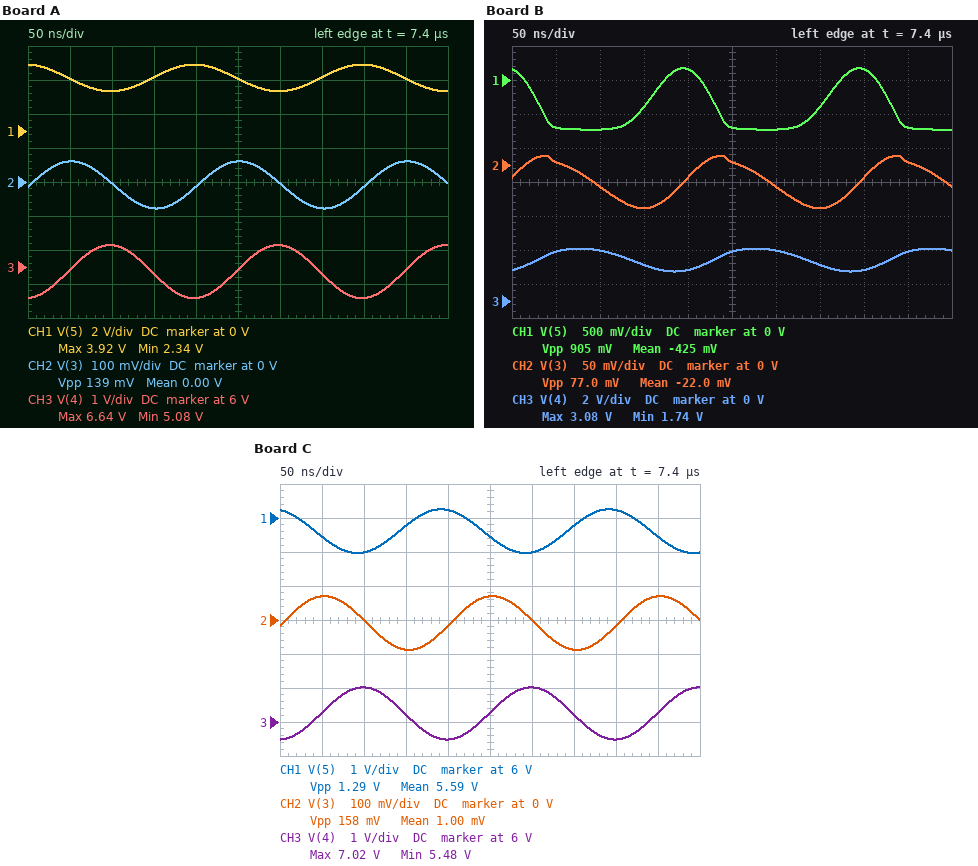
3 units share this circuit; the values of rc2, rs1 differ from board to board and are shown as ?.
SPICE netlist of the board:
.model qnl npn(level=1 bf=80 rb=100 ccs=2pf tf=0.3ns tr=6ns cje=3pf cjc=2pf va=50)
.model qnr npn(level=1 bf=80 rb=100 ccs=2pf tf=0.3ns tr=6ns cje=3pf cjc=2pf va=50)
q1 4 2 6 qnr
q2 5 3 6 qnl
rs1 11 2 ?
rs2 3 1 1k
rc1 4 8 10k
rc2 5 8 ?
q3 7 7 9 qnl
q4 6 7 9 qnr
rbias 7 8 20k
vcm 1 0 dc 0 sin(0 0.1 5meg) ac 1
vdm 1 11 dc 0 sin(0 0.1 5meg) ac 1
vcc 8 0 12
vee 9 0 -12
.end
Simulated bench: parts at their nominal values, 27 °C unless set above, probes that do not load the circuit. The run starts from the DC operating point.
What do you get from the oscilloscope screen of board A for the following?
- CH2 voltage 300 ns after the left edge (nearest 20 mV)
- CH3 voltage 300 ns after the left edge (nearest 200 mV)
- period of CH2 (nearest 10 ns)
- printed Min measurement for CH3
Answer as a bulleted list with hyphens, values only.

- 0 V
- 6.6 V
- 200 ns
- 5.08 V
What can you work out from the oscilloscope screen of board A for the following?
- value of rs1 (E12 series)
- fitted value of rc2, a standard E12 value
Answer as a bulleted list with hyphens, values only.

- 2.2 kΩ
- 12 kΩ
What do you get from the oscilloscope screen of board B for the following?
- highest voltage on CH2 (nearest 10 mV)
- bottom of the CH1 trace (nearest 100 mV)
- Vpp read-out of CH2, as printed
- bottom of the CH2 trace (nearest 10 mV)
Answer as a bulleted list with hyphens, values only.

- 10 mV
- -700 mV
- 77.0 mV
- -60 mV
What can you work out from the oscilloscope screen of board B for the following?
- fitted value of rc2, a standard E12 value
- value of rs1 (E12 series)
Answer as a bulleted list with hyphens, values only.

- 33 kΩ
- 680 Ω
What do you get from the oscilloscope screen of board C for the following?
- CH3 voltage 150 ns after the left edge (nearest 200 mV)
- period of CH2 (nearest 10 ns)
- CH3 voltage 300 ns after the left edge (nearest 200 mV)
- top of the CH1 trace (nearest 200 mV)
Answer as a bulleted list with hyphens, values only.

- 6.2 V
- 200 ns
- 7.0 V
- 6.2 V
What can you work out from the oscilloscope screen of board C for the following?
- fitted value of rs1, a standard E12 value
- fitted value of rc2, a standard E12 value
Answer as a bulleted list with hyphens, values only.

- 2.7 kΩ
- 8.2 kΩ
